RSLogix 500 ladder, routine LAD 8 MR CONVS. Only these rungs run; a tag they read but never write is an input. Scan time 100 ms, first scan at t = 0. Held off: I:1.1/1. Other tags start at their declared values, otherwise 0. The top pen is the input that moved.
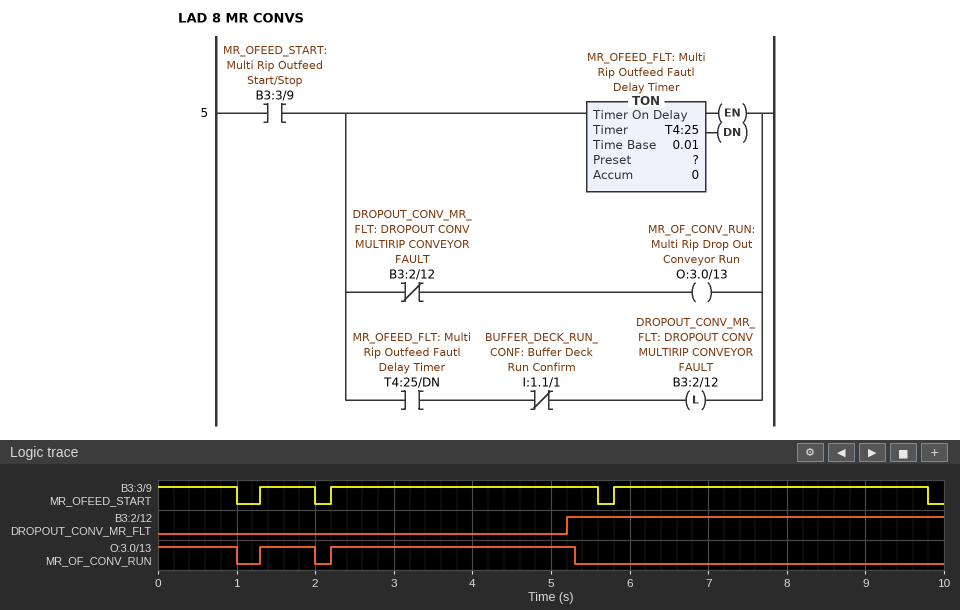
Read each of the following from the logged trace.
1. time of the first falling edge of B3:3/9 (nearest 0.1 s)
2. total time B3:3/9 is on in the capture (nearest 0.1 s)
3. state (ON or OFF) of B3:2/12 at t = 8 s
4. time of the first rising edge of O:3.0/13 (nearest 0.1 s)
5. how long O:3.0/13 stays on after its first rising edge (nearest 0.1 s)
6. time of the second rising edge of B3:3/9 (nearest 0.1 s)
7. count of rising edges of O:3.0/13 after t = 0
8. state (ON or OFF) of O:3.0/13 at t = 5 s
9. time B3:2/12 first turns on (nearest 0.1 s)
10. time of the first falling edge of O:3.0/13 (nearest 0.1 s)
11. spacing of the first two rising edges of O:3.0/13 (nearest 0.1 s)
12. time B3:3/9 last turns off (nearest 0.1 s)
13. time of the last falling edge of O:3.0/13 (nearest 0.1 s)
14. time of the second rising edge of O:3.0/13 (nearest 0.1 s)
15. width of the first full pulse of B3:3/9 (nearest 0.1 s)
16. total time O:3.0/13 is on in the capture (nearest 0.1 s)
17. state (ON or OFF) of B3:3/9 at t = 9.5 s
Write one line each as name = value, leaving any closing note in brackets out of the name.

time of the first falling edge of B3:3/9 = 1.0 s
total time B3:3/9 is on in the capture = 9.1 s
state (ON or OFF) of B3:2/12 at t = 8 s = ON
time of the first rising edge of O:3.0/13 = 1.3 s
how long O:3.0/13 stays on after its first rising edge = 0.7 s
time of the second rising edge of B3:3/9 = 2.2 s
count of rising edges of O:3.0/13 after t = 0 = 2
state (ON or OFF) of O:3.0/13 at t = 5 s = ON
time B3:2/12 first turns on = 5.2 s
time of the first falling edge of O:3.0/13 = 1.0 s
spacing of the first two rising edges of O:3.0/13 = 0.9 s
time B3:3/9 last turns off = 9.8 s
time of the last falling edge of O:3.0/13 = 5.3 s
time of the second rising edge of O:3.0/13 = 2.2 s
width of the first full pulse of B3:3/9 = 0.7 s
total time O:3.0/13 is on in the capture = 4.8 s
state (ON or OFF) of B3:3/9 at t = 9.5 s = ON
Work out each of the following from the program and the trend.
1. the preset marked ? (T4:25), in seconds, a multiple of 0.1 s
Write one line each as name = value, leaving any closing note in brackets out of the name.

the preset marked ? (T4:25), in seconds, a multiple of 0.1 s = 3.0 s
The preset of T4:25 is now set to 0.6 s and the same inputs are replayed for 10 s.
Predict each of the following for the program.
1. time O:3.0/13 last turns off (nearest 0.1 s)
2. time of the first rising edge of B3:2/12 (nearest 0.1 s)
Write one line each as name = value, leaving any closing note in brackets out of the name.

time O:3.0/13 last turns off = 0.7 s
time of the first rising edge of B3:2/12 = 0.6 s
